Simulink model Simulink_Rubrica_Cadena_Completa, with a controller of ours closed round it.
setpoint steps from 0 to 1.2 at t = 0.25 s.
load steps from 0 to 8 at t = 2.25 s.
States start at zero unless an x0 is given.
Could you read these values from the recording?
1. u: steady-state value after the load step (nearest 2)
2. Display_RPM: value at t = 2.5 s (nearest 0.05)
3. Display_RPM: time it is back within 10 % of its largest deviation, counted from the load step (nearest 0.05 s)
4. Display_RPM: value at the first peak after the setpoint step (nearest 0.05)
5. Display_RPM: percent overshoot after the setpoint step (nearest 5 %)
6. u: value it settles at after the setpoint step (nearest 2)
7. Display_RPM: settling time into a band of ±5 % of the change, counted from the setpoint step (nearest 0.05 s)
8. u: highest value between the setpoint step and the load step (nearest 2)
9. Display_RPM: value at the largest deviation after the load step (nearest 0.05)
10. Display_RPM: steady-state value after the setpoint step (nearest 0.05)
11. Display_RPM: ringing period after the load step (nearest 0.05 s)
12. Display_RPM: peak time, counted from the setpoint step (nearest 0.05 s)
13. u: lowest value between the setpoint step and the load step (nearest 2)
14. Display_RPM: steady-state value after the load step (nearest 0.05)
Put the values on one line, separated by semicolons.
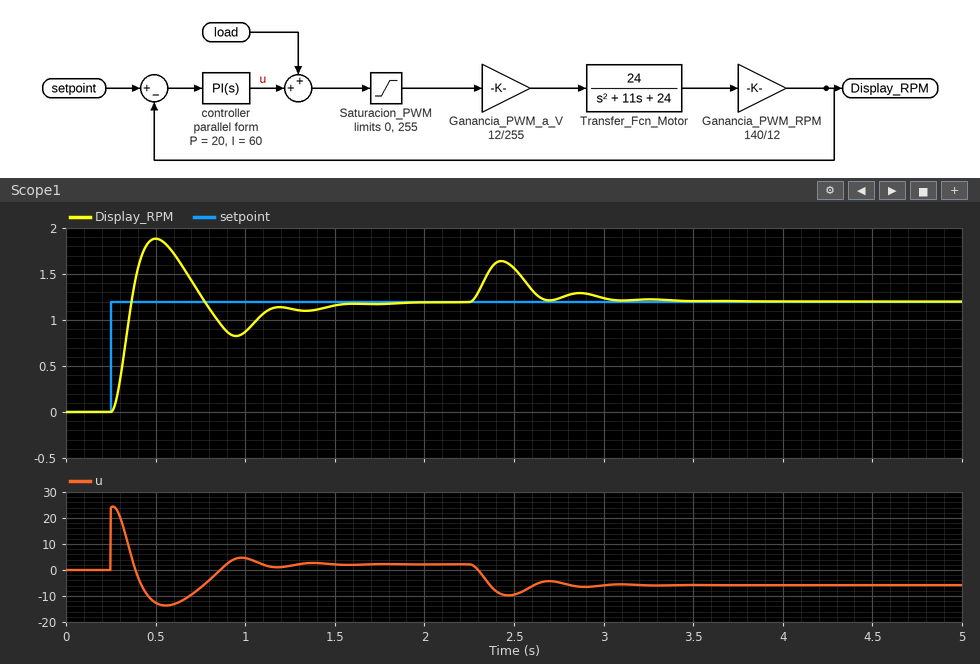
-6; 1.55; 0.75 s; 1.90; 55 %; 2; 1.20 s; 24; 1.65; 1.20; 0.45 s; 0.25 s; -14; 1.20
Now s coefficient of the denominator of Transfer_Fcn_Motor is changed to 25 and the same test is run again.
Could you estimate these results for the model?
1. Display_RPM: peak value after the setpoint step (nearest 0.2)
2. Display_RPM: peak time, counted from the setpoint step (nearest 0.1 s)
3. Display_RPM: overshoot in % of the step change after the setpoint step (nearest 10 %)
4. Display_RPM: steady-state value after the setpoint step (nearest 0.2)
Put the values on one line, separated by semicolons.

1.4; 0.3 s; 20 %; 1.2
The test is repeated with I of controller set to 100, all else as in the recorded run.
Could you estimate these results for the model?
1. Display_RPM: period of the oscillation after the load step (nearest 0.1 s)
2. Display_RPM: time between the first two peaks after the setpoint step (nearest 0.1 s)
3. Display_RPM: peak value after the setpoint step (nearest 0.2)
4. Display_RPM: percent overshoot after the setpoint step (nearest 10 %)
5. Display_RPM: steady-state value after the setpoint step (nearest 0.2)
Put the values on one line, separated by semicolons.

0.5 s; 0.8 s; 2.0; 70 %; 1.2
